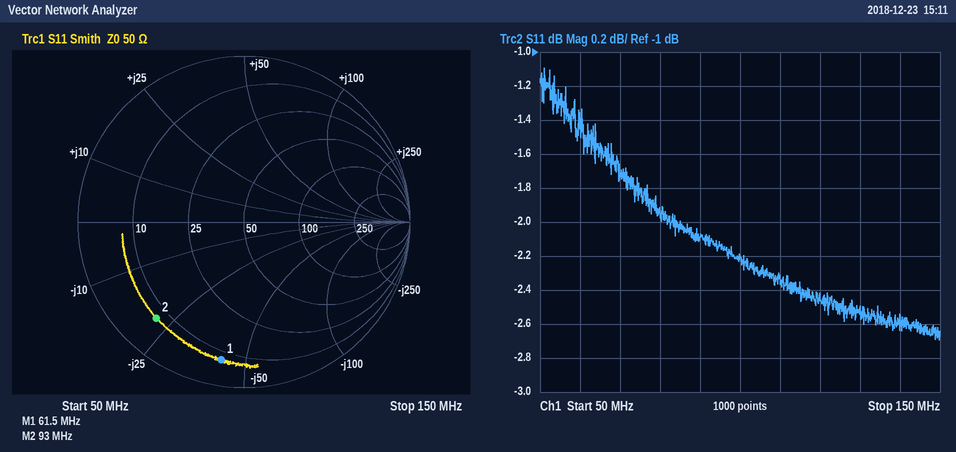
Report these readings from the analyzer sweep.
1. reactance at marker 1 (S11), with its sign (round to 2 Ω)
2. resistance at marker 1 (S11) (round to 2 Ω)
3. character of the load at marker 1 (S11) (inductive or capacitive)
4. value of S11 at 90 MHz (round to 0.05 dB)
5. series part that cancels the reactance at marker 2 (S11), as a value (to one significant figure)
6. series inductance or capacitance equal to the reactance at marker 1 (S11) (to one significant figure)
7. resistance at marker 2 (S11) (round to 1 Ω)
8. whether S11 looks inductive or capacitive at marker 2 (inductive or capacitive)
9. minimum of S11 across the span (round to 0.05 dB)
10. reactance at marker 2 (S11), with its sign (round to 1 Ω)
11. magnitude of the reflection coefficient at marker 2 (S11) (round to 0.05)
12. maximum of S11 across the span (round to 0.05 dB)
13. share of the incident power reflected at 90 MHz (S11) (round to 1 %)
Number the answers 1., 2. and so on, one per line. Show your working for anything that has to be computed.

1. -42 Ω
2. 8 Ω
3. capacitive
4. -2.10 dB
5. L = 22 Ω/(2π × 93 MHz) ≈ 37.6 nH, so 40 nH to one significant figure
6. C = 1/(2π × 61.5 MHz × 42 Ω) ≈ 61.6 pF, so 60 pF to one significant figure
7. 7 Ω
8. capacitive
9. -2.70 dB
10. -22 Ω
11. 0.80
12. -1.10 dB
13. 10^(-2.1/10) ≈ 62 %
